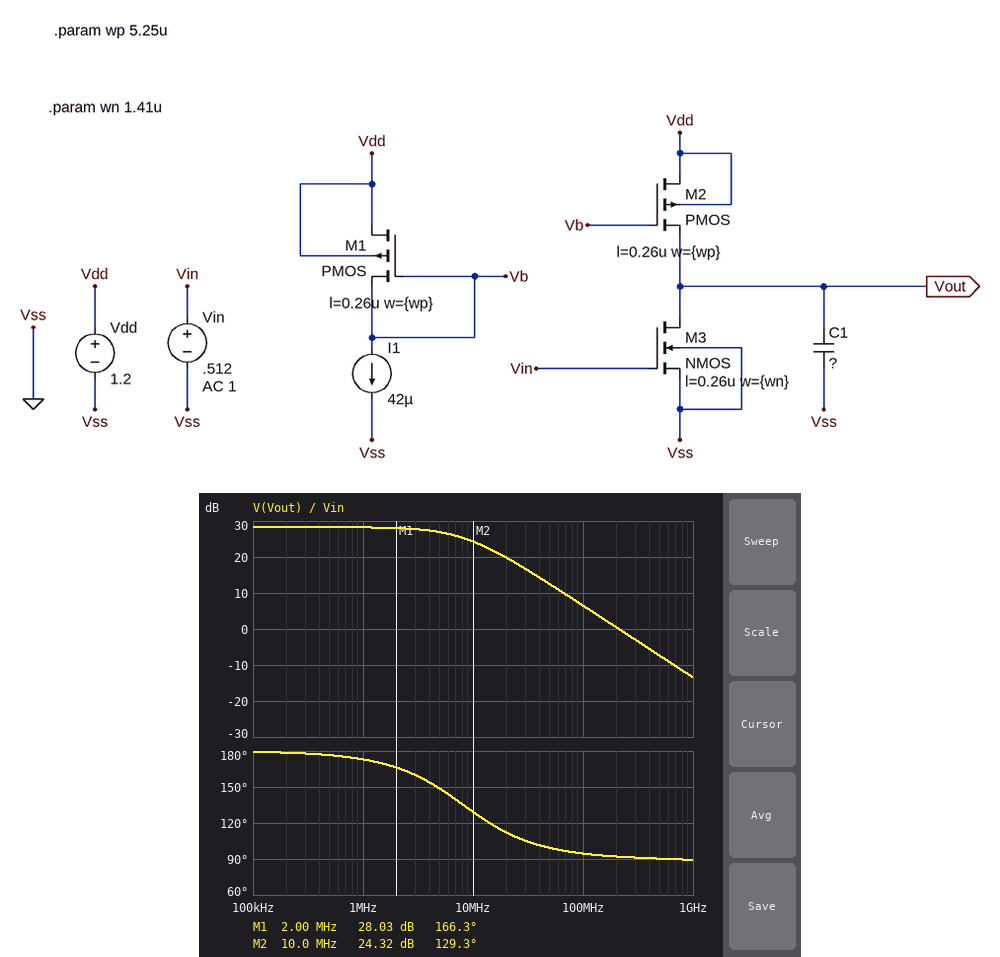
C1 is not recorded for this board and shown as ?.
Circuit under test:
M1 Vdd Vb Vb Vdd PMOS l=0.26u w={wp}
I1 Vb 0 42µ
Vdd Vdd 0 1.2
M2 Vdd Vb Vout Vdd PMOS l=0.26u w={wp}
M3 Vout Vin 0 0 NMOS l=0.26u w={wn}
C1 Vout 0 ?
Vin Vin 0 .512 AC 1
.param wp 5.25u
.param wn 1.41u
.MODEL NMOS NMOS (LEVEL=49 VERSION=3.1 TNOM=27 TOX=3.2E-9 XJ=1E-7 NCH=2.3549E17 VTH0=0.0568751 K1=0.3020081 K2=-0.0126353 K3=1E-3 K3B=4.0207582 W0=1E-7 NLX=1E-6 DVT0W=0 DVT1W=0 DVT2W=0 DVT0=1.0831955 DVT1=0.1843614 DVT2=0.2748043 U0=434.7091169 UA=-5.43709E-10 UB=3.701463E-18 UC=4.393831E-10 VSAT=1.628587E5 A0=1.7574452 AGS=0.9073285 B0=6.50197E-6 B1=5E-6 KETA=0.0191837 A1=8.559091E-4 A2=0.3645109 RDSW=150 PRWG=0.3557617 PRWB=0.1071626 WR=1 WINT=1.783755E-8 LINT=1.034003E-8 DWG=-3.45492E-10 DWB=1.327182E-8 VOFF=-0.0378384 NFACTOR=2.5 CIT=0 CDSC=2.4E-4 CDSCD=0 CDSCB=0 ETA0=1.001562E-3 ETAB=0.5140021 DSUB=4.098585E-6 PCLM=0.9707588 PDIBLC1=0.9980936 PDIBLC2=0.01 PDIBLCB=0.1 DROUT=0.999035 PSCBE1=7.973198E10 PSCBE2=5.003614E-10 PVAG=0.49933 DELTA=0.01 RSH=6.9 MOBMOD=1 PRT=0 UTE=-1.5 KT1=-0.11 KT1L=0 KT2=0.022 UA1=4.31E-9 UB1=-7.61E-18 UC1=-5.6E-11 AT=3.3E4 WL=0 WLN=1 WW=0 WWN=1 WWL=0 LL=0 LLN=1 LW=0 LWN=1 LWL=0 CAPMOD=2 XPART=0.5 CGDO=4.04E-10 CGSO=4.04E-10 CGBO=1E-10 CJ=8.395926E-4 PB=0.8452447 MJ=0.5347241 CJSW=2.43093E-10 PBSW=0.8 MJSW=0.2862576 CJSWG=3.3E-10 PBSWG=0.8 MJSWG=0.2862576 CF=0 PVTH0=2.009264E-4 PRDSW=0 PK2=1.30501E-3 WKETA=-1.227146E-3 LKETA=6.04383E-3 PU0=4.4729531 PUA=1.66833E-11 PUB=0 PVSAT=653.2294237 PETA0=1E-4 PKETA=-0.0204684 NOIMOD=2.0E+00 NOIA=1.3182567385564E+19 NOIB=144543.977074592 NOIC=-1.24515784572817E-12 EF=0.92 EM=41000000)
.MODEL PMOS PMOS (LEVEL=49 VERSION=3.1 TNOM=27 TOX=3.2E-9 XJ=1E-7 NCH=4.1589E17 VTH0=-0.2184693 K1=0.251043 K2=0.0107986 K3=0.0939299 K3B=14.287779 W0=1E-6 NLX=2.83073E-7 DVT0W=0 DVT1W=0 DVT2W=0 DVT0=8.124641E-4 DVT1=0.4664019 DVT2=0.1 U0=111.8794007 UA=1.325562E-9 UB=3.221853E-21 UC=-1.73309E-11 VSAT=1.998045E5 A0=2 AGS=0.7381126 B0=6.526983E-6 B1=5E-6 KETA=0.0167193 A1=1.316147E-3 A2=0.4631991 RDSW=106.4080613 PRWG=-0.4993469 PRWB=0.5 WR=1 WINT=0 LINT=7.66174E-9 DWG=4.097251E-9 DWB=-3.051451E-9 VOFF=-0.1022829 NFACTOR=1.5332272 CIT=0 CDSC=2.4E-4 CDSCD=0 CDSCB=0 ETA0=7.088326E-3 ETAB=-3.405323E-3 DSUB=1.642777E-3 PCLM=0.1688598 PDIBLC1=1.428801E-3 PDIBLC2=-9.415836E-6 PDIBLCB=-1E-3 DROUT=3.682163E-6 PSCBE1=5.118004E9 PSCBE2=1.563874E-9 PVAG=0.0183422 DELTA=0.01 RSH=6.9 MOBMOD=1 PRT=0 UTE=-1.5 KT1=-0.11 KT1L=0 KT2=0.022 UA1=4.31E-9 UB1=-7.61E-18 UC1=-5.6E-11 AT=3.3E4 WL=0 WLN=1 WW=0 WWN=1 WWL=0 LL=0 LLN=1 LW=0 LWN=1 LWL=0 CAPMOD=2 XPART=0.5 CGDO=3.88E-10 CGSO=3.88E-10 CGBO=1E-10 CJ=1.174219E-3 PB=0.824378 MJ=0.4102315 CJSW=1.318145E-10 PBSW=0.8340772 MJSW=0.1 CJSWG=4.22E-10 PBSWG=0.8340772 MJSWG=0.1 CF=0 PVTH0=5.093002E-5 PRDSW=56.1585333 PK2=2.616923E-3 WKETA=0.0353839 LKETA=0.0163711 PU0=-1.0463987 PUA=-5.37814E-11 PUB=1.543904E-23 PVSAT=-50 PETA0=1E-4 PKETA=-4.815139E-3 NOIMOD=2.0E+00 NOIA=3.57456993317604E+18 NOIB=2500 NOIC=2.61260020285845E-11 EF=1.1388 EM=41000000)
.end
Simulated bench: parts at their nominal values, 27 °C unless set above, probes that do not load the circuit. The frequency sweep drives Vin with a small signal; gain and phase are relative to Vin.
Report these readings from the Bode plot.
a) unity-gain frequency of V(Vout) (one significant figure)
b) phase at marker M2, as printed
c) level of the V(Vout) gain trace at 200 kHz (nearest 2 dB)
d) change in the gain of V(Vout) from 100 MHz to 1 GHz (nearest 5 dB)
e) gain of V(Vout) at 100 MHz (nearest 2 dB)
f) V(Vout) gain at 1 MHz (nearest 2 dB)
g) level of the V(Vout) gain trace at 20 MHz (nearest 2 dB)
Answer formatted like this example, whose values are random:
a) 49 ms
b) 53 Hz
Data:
a) 200 MHz
b) 129.3 deg
c) 28 dB
d) -20 dB
e) 6 dB
f) 28 dB
g) 20 dB
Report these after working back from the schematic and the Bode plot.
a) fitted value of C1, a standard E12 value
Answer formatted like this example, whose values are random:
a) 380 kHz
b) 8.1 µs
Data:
a) 330 fF
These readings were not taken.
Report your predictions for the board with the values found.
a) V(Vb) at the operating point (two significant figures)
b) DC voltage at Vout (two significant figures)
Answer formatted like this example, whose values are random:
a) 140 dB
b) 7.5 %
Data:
a) 670 mV
b) 620 mV
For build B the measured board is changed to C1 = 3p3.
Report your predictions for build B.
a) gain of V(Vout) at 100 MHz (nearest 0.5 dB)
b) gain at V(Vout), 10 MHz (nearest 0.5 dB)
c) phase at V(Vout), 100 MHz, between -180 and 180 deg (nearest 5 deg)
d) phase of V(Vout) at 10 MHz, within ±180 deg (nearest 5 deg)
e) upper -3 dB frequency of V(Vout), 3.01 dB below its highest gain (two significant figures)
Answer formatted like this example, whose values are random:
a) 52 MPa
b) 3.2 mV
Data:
a) -13.5 dB
b) 6.5 dB
c) 90 deg
d) 95 deg
e) 830 kHz
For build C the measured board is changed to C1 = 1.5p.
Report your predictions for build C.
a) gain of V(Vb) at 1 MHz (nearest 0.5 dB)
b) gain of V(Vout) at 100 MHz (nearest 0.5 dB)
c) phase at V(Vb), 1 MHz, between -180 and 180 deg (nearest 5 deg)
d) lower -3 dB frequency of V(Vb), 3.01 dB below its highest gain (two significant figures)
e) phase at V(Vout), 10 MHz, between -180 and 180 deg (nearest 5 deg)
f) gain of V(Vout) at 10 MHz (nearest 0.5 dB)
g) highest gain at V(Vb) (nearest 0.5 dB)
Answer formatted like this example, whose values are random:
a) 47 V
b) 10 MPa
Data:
a) -63.0 dB
b) -6.5 dB
c) -120 deg
d) 1.8 MHz
e) 100 deg
f) 13.5 dB
g) -56.5 dB
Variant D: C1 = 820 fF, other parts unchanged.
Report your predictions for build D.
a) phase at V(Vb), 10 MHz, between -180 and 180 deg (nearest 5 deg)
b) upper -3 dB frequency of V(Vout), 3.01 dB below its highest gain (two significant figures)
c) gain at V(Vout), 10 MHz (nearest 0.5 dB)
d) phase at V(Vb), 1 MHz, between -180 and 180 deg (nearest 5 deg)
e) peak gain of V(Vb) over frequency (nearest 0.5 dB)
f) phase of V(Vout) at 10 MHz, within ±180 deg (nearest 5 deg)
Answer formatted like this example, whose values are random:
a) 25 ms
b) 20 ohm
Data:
a) -160 deg
b) 3.3 MHz
c) 18.5 dB
d) -105 deg
e) -51.5 dB
f) 110 deg
